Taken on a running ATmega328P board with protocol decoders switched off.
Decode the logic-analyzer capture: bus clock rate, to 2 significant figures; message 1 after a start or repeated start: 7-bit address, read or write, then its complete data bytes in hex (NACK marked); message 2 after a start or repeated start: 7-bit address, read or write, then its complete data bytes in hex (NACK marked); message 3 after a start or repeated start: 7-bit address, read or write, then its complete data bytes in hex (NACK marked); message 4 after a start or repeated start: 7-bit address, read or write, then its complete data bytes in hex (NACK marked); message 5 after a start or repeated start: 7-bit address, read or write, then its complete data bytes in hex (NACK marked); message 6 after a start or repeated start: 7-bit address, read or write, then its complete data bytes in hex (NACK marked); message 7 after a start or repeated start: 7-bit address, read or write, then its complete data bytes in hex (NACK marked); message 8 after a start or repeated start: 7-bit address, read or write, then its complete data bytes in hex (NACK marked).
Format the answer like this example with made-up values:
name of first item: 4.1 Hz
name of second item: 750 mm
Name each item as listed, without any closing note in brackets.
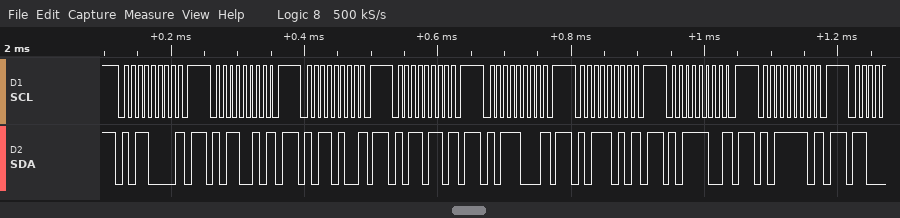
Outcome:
bus clock rate, to 2 significant figures: 100 kHz
message 1 after a start or repeated start: 7-bit address, read or write, then its complete data bytes in hex: 0x58 write NACK
message 2 after a start or repeated start: 7-bit address, read or write, then its complete data bytes in hex: 0x59 write NACK
message 3 after a start or repeated start: 7-bit address, read or write, then its complete data bytes in hex: 0x5A write NACK
message 4 after a start or repeated start: 7-bit address, read or write, then its complete data bytes in hex: 0x5B write NACK
message 5 after a start or repeated start: 7-bit address, read or write, then its complete data bytes in hex: 0x5C write NACK
message 6 after a start or repeated start: 7-bit address, read or write, then its complete data bytes in hex: 0x5D write NACK
message 7 after a start or repeated start: 7-bit address, read or write, then its complete data bytes in hex: 0x5E write NACK
message 8 after a start or repeated start: 7-bit address, read or write, then its complete data bytes in hex: 0x5F write NACK
